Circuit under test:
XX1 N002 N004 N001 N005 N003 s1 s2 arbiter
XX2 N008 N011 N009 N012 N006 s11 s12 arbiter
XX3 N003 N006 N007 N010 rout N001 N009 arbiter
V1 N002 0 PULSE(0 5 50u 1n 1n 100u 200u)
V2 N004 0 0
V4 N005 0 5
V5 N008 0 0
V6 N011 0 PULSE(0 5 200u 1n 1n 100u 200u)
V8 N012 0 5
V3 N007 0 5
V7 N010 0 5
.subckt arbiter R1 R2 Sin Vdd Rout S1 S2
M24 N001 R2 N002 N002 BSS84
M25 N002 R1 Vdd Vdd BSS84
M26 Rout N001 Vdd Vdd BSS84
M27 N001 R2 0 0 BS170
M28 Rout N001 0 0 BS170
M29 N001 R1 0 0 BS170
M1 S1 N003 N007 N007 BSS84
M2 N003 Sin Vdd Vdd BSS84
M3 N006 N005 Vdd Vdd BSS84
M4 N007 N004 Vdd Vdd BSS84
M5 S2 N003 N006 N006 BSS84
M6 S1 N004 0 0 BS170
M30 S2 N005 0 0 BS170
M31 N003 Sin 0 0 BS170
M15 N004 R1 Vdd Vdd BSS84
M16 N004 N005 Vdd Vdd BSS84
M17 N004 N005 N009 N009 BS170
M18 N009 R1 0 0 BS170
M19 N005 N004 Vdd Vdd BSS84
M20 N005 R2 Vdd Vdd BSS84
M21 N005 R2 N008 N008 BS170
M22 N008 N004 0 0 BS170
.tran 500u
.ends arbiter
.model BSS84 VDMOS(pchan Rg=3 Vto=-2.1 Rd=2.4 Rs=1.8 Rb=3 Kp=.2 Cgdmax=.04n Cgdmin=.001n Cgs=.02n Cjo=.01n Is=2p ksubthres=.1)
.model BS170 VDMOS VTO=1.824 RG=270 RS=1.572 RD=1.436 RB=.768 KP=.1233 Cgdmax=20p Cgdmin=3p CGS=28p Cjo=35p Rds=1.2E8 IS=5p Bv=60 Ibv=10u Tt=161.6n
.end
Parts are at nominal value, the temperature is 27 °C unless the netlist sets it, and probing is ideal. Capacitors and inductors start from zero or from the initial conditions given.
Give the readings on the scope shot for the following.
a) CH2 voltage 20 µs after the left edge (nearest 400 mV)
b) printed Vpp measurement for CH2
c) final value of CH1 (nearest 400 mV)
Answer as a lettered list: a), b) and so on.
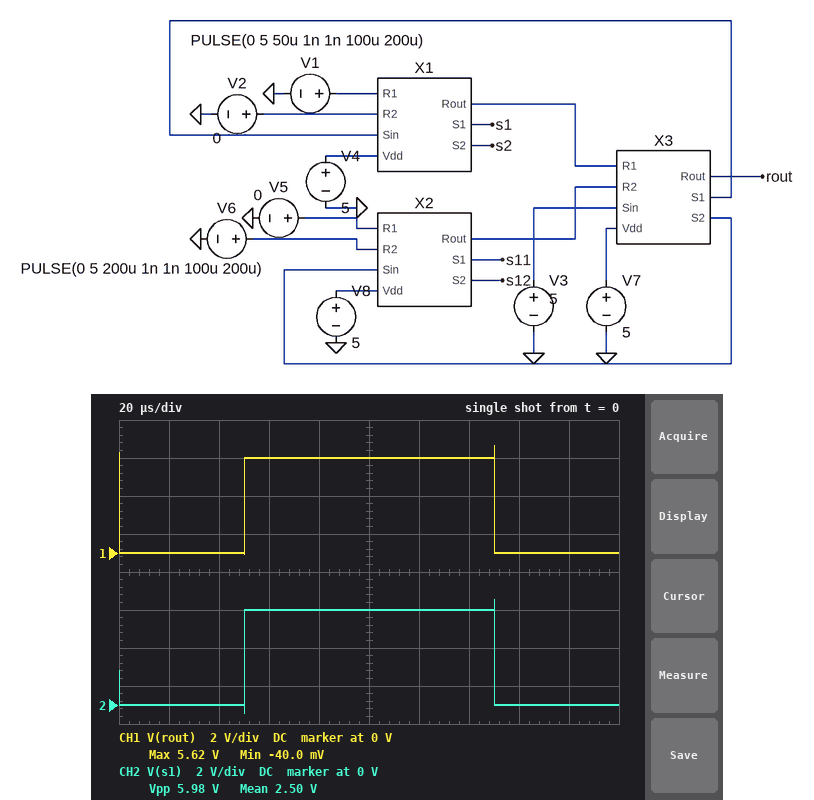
a) 0 V
b) 5.98 V
c) 0 V
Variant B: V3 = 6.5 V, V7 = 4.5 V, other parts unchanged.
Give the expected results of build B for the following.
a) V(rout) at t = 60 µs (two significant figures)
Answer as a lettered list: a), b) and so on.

a) 4.5 V
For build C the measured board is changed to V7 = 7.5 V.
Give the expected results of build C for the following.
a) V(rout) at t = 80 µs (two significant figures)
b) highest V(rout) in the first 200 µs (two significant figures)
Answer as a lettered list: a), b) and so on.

a) 7.5 V
b) 7.6 V
